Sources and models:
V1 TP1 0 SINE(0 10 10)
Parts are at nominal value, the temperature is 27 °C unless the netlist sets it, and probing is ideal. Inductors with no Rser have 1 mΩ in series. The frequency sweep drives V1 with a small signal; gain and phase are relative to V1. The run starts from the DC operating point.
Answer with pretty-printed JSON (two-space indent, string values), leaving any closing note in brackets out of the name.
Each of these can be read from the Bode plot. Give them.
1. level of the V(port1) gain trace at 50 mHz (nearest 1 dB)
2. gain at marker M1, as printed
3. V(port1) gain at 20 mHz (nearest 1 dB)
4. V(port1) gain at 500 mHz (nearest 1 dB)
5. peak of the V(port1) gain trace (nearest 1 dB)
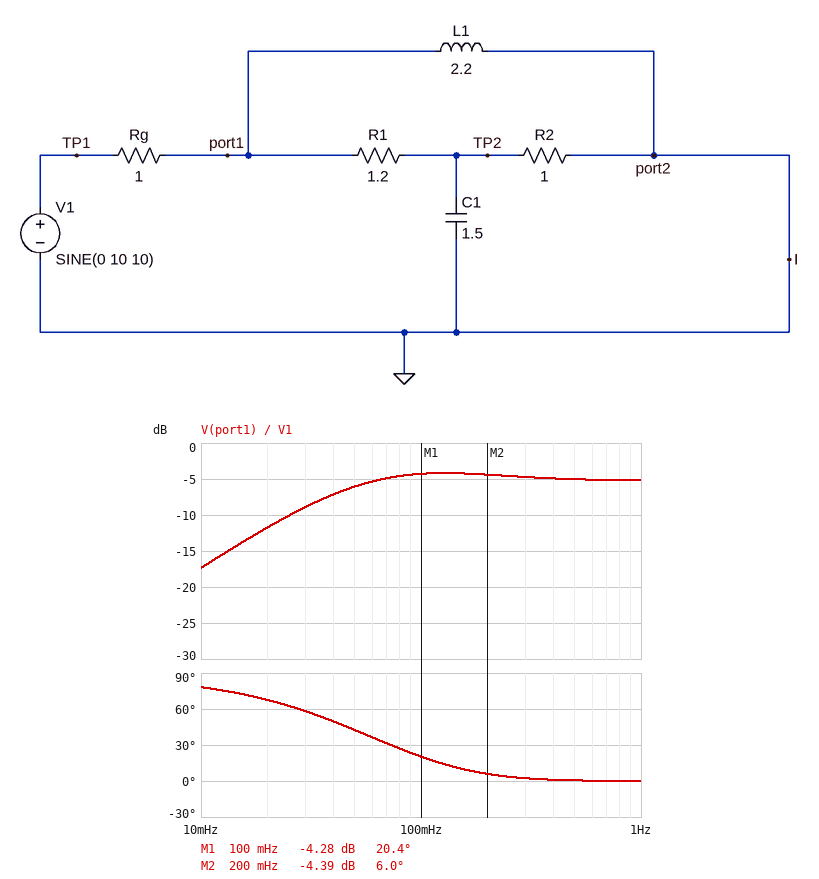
{
  "level of the V(port1) gain trace at 50 mHz": "-6 dB",
  "gain at marker M1, as printed": "-4.28 dB",
  "V(port1) gain at 20 mHz": "-12 dB",
  "V(port1) gain at 500 mHz": "-5 dB",
  "peak of the V(port1) gain trace": "-4 dB"
}
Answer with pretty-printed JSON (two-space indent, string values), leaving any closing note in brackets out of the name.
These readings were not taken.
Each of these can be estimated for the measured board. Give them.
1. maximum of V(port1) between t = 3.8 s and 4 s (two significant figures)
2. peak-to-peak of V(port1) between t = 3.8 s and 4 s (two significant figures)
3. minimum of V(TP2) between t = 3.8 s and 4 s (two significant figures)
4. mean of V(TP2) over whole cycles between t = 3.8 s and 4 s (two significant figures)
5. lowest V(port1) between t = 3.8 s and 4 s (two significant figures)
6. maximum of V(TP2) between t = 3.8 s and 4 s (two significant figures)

{
  "maximum of V(port1) between t = 3.8 s and 4 s": "5.4 V",
  "peak-to-peak of V(port1) between t = 3.8 s and 4 s": "11 V",
  "minimum of V(TP2) between t = 3.8 s and 4 s": "-54 mV",
  "mean of V(TP2) over whole cycles between t = 3.8 s and 4 s": "-5.6 mV",
  "lowest V(port1) between t = 3.8 s and 4 s": "-5.5 V",
  "maximum of V(TP2) between t = 3.8 s and 4 s": "43 mV"
}
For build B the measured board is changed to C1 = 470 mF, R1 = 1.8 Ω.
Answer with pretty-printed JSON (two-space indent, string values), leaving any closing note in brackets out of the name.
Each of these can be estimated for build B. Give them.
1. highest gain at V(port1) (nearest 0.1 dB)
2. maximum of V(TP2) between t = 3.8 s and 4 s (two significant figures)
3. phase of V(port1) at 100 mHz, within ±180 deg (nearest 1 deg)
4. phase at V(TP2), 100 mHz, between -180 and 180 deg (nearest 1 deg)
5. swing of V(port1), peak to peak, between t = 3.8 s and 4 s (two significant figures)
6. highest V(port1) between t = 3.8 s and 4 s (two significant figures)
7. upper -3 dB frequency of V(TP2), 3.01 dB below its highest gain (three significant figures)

{
  "highest gain at V(port1)": "-3.0 dB",
  "maximum of V(TP2) between t = 3.8 s and 4 s": "120 mV",
  "phase of V(port1) at 100 mHz, within ±180 deg": "27 deg",
  "phase at V(TP2), 100 mHz, between -180 and 180 deg": "16 deg",
  "swing of V(port1), peak to peak, between t = 3.8 s and 4 s": "13 V",
  "highest V(port1) between t = 3.8 s and 4 s": "6.4 V",
  "upper -3 dB frequency of V(TP2), 3.01 dB below its highest gain": "551 mHz"
}
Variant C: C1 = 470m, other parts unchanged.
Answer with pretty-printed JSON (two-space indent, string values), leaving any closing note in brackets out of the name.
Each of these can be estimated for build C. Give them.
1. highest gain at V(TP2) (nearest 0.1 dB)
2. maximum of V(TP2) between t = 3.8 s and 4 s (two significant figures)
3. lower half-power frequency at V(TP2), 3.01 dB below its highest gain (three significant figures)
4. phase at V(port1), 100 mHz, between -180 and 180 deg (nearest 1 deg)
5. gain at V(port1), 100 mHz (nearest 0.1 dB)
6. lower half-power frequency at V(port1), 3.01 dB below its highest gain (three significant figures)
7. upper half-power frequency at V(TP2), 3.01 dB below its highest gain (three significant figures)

{
  "highest gain at V(TP2)": "-10.8 dB",
  "maximum of V(TP2) between t = 3.8 s and 4 s": "150 mV",
  "lower half-power frequency at V(TP2), 3.01 dB below its highest gain": "42.7 mHz",
  "phase at V(port1), 100 mHz, between -180 and 180 deg": "24 deg",
  "gain at V(port1), 100 mHz": "-4.1 dB",
  "lower half-power frequency at V(port1), 3.01 dB below its highest gain": "45.5 mHz",
  "upper half-power frequency at V(TP2), 3.01 dB below its highest gain": "575 mHz"
}
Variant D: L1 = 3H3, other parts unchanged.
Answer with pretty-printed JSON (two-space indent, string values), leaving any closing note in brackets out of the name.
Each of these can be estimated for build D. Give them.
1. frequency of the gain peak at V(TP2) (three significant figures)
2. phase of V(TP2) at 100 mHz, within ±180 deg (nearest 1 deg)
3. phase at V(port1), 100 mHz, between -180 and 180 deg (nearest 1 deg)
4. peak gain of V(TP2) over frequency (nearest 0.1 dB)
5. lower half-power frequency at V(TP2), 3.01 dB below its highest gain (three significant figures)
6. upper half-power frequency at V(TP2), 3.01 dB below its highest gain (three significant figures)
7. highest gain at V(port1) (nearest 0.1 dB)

{
  "frequency of the gain peak at V(TP2)": "71.6 mHz",
  "phase of V(TP2) at 100 mHz, within ±180 deg": "-15 deg",
  "phase at V(port1), 100 mHz, between -180 and 180 deg": "12 deg",
  "peak gain of V(TP2) over frequency": "-11.5 dB",
  "lower half-power frequency at V(TP2), 3.01 dB below its highest gain": "24.9 mHz",
  "upper half-power frequency at V(TP2), 3.01 dB below its highest gain": "206 mHz",
  "highest gain at V(port1)": "-3.9 dB"
}
